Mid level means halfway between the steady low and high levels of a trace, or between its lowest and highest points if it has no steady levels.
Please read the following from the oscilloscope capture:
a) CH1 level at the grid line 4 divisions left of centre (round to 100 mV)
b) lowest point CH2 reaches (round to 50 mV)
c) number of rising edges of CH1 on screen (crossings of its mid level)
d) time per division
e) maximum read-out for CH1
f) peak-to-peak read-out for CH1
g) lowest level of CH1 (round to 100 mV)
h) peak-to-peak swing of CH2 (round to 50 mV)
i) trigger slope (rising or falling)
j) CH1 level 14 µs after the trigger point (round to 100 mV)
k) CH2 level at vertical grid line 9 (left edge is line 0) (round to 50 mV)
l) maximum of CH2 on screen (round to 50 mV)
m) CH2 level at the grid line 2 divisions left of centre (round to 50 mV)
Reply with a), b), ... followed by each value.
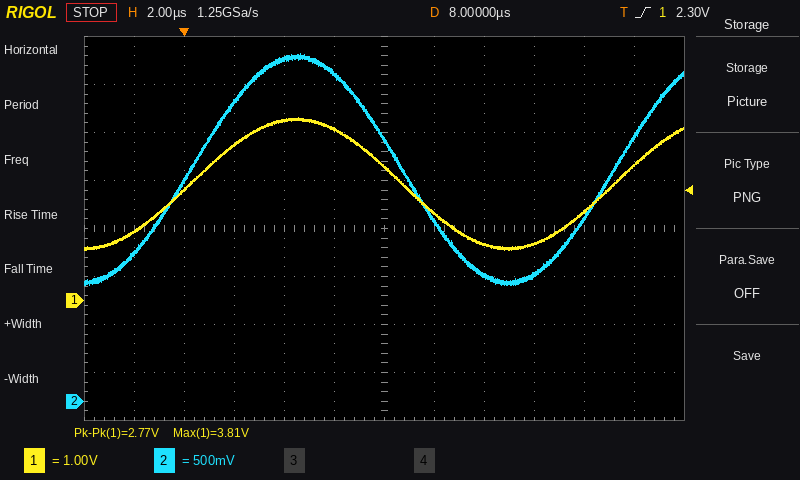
a) 2.3 V
b) 1.20 V
c) 2
d) 2 µs
e) 3.81 V
f) 2.77 V
g) 1.0 V
h) 2.40 V
i) rising
j) 1.2 V
k) 1.30 V
l) 3.60 V
m) 3.55 V
